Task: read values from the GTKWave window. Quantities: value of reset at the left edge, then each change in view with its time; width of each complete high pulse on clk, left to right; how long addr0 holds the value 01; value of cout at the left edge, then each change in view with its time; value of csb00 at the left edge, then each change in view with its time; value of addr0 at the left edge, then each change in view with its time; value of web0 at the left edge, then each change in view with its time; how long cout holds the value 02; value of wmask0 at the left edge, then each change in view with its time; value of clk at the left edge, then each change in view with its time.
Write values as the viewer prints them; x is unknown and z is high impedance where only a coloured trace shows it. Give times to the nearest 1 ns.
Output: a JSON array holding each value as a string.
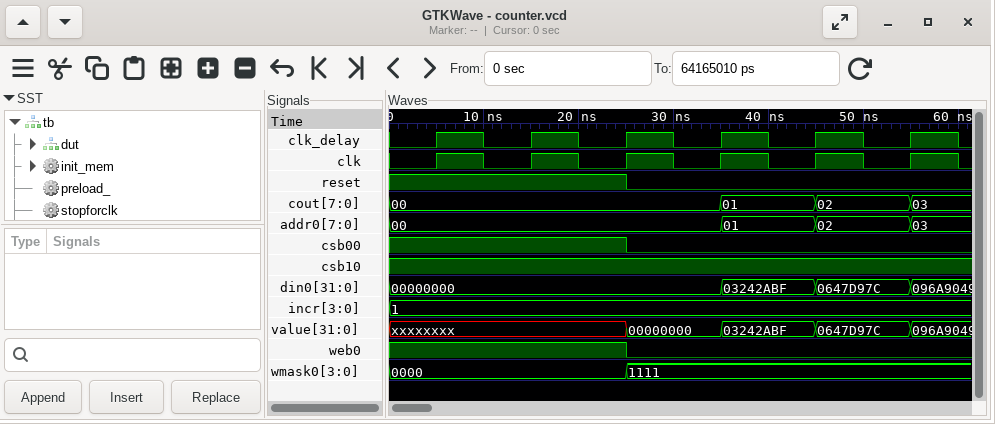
["1, 0 at 25 ns", "5 ns, 5 ns, 5 ns, 5 ns, 5 ns, 5 ns", "10 ns", "00, 01 at 35 ns, 02 at 45 ns, 03 at 55 ns", "1, 0 at 25 ns", "00, 01 at 35 ns, 02 at 45 ns, 03 at 55 ns", "1, 0 at 25 ns", "10 ns", "0000, 1111 at 25 ns", "0, 1 at 5 ns, 0 at 10 ns, 1 at 15 ns, 0 at 20 ns, 1 at 25 ns, 0 at 30 ns, 1 at 35 ns, 0 at 40 ns, 1 at 45 ns, 0 at 50 ns, 1 at 55 ns, 0 at 60 ns"]
